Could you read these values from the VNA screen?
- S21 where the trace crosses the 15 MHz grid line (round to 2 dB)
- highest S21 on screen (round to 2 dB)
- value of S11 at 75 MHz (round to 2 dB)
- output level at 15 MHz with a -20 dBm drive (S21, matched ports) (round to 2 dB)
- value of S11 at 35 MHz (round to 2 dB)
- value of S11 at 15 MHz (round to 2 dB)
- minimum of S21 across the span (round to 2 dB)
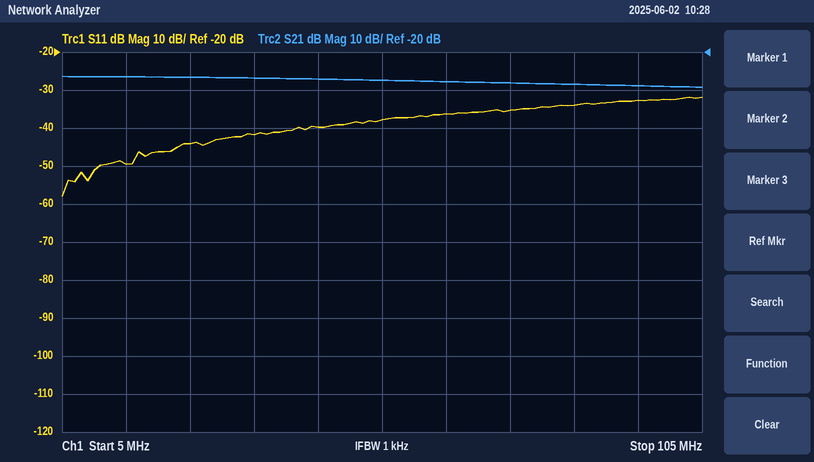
-26 dB
-26 dB
-36 dB
-46 dBm
-42 dB
-50 dB
-30 dB
